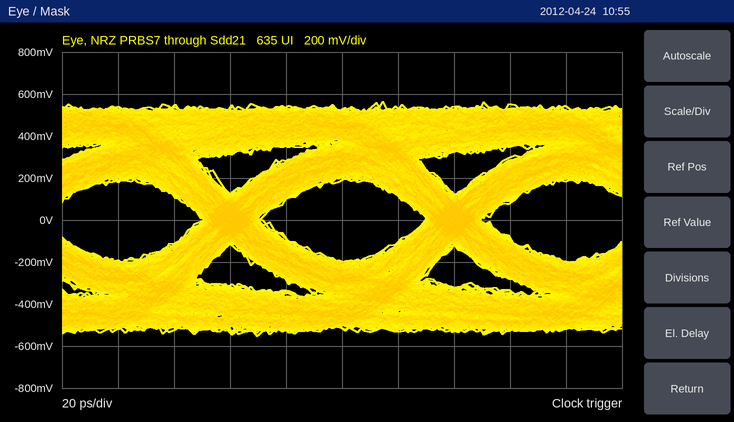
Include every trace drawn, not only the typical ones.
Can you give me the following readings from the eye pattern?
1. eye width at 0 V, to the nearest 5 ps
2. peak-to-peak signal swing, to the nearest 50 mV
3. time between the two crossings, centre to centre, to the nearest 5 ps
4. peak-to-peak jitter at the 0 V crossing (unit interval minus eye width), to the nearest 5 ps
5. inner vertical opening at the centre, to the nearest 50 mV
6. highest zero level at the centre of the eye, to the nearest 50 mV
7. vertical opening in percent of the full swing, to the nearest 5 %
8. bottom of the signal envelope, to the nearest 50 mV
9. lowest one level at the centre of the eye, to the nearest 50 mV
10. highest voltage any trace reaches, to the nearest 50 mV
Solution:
60 ps
1.10 V
80 ps
20 ps
400 mV
-200 mV
35 %
-550 mV
200 mV
550 mV
